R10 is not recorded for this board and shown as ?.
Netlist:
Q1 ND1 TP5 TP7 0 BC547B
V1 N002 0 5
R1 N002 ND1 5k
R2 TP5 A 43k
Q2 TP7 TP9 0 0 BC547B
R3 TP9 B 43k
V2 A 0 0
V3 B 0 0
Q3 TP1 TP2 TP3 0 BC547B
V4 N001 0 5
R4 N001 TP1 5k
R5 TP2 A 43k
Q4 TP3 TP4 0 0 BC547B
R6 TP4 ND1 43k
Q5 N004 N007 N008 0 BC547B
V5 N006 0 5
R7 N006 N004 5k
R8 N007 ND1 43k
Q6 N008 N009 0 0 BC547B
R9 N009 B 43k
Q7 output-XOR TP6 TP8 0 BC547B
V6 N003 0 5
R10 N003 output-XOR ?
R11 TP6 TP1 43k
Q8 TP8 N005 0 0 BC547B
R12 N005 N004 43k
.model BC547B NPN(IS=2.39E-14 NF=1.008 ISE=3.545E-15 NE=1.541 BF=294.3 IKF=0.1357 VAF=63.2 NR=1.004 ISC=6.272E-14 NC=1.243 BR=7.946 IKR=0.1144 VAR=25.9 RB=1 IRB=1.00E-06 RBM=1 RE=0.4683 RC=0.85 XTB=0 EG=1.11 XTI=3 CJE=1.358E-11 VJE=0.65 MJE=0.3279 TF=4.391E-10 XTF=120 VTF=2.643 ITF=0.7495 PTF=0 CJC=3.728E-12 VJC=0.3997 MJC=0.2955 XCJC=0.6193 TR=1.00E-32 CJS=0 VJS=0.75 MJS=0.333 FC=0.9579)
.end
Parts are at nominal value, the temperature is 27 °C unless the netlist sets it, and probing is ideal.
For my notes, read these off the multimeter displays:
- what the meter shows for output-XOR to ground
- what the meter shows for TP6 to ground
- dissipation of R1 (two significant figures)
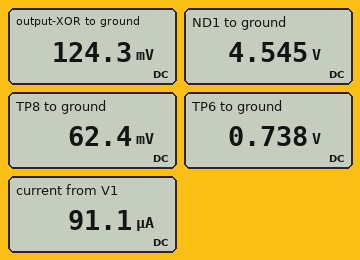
124.3 mV
0.738 V
41 µW
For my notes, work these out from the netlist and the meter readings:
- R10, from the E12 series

1.5 kΩ
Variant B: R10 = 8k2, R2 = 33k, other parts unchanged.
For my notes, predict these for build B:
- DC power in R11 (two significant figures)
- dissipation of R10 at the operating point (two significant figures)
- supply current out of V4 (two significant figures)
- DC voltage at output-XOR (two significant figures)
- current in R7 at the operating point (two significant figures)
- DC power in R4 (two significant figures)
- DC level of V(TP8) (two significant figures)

350 µW
3.0 mW
90 µA
52 mV
91 µA
41 µW
27 mV
